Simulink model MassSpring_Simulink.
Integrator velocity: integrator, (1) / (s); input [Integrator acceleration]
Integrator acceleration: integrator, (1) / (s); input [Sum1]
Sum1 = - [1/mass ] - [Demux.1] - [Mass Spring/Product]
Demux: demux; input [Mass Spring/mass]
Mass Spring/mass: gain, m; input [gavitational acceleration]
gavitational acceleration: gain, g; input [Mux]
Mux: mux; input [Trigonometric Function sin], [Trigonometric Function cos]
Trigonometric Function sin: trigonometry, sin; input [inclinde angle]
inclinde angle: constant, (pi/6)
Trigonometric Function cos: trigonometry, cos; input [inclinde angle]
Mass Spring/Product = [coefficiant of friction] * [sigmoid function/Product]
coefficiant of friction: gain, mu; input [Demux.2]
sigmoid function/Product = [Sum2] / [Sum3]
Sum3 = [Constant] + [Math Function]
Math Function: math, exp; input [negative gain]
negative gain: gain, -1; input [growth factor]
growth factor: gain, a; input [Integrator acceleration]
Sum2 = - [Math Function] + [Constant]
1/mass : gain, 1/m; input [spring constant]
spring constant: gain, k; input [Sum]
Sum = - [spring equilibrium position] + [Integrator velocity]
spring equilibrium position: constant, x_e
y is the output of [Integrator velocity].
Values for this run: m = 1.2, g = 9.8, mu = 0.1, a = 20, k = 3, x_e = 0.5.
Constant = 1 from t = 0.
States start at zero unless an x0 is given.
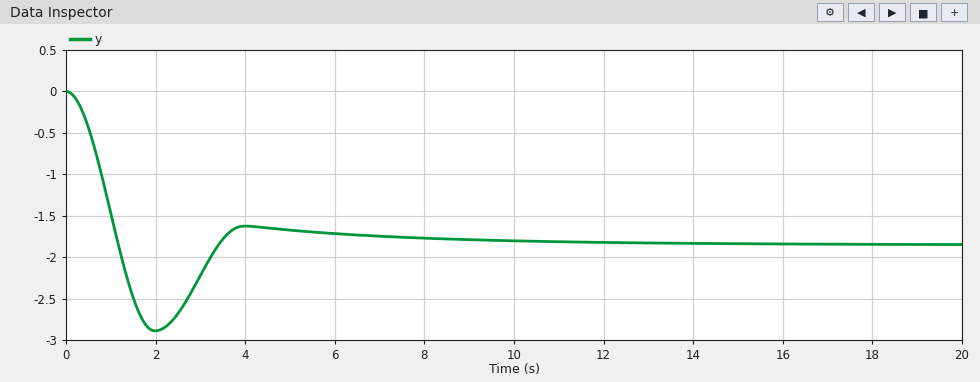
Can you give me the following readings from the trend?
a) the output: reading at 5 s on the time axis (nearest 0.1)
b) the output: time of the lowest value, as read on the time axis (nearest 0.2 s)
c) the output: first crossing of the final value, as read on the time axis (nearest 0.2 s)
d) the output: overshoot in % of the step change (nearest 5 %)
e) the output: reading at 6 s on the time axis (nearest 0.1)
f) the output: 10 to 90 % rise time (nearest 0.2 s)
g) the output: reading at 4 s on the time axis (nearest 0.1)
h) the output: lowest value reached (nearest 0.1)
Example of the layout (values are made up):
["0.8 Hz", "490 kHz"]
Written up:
["-1.7", "2.0 s", "1.2 s", "55 %", "-1.7", "0.8 s", "-1.6", "-2.9"]
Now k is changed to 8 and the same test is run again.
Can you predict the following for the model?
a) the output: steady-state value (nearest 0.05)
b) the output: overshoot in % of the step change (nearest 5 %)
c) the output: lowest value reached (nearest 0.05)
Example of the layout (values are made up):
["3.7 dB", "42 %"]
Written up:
["-0.40", "20 %", "-0.45"]
